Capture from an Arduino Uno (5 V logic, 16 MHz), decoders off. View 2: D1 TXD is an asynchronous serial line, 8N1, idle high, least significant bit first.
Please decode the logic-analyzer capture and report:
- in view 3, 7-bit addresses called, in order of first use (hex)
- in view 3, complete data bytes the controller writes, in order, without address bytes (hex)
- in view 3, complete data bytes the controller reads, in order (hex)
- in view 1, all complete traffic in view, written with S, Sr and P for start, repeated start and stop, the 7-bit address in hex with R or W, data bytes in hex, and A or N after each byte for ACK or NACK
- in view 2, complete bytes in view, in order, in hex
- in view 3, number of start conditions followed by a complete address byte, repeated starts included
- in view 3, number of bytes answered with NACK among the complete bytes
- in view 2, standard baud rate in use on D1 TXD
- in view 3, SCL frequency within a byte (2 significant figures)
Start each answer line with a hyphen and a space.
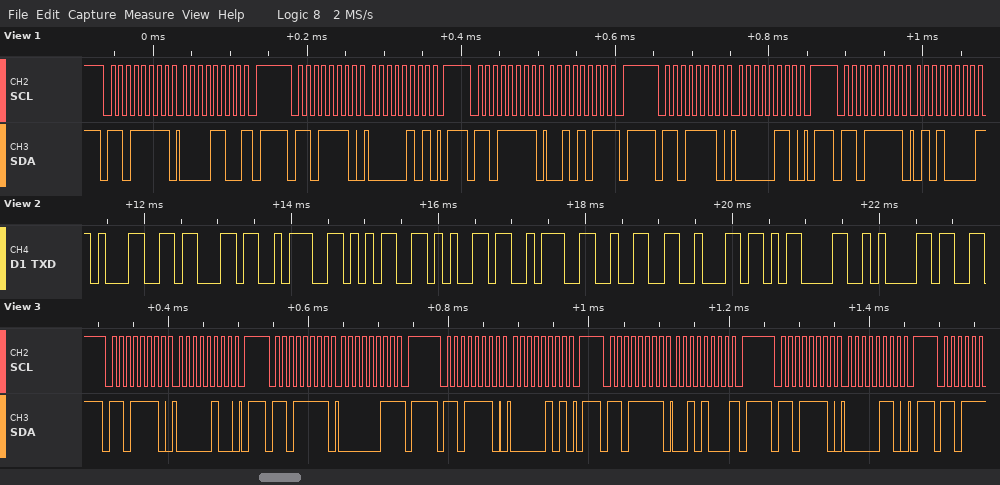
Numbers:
- 0x6F
- 04 05 06
- 03 28
- S 6FR A 0C N P S 6FW A 05 A P S 6FR A 2B N P S 6FW A 06 A P S 6FR A 50 N
- 31 63 3A 35 65 3A 32 62 0D 0A
- 5
- 2
- 9600 baud
- 100 kHz
